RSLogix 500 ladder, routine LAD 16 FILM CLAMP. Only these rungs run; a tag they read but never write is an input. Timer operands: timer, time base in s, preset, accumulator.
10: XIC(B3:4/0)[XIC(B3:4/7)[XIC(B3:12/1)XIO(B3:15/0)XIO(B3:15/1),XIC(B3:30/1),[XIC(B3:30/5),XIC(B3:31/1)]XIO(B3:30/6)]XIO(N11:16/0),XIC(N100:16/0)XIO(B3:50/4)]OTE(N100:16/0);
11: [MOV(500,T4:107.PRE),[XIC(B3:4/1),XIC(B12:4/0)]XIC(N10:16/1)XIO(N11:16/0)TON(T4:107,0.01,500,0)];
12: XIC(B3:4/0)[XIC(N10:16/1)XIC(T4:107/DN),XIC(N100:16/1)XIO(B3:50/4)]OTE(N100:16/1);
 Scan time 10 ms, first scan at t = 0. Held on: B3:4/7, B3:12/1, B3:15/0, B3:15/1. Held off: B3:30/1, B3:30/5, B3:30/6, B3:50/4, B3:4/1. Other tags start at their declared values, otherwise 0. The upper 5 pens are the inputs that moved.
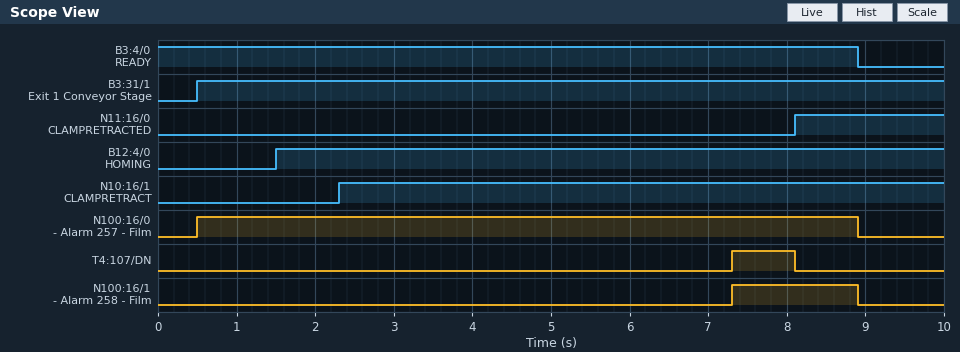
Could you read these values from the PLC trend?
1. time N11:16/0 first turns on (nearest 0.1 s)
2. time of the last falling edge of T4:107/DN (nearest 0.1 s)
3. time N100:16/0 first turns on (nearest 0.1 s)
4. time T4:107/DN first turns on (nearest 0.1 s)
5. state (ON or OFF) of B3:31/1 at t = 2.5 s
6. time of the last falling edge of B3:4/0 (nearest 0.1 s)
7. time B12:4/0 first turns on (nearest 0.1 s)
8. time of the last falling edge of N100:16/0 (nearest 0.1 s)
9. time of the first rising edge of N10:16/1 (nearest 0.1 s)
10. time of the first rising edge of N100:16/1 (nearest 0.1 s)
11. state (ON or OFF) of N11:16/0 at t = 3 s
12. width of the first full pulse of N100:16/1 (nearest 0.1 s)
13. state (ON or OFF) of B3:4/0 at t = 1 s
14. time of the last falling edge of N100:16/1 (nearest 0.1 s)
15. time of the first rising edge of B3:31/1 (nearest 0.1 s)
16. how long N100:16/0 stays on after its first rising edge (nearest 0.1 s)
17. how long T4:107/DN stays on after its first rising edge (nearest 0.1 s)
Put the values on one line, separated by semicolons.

8.1 s; 8.1 s; 0.5 s; 7.3 s; ON; 8.9 s; 1.5 s; 8.9 s; 2.3 s; 7.3 s; OFF; 1.6 s; ON; 8.9 s; 0.5 s; 8.4 s; 0.8 s
